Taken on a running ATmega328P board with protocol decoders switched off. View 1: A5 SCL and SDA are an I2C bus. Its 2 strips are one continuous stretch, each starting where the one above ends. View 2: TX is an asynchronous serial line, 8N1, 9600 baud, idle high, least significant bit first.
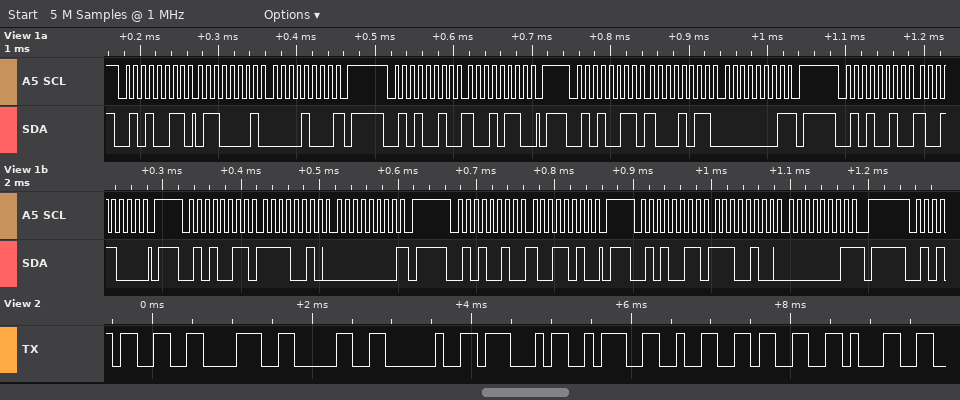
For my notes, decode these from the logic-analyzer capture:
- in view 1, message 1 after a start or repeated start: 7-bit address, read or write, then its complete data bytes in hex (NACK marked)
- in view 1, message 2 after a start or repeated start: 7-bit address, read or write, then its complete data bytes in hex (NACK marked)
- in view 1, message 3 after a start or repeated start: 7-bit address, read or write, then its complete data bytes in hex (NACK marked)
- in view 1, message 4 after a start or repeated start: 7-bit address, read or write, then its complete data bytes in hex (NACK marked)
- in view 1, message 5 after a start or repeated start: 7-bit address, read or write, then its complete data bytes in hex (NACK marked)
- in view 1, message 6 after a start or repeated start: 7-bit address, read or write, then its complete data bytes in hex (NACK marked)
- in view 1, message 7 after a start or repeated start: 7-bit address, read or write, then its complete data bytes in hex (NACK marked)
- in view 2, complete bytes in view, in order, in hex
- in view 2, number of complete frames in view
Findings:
0x29 read: 61 08 NACK
0x29 write: 96
0x29 read: 8B 01 NACK
0x29 write: 98
0x29 read: F2 00 NACK
0x29 write: 9A
0x29 read: E4 01 NACK
33 38 30 20 47 3A 32 33 31
9
